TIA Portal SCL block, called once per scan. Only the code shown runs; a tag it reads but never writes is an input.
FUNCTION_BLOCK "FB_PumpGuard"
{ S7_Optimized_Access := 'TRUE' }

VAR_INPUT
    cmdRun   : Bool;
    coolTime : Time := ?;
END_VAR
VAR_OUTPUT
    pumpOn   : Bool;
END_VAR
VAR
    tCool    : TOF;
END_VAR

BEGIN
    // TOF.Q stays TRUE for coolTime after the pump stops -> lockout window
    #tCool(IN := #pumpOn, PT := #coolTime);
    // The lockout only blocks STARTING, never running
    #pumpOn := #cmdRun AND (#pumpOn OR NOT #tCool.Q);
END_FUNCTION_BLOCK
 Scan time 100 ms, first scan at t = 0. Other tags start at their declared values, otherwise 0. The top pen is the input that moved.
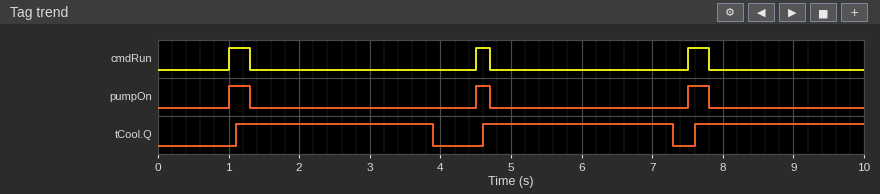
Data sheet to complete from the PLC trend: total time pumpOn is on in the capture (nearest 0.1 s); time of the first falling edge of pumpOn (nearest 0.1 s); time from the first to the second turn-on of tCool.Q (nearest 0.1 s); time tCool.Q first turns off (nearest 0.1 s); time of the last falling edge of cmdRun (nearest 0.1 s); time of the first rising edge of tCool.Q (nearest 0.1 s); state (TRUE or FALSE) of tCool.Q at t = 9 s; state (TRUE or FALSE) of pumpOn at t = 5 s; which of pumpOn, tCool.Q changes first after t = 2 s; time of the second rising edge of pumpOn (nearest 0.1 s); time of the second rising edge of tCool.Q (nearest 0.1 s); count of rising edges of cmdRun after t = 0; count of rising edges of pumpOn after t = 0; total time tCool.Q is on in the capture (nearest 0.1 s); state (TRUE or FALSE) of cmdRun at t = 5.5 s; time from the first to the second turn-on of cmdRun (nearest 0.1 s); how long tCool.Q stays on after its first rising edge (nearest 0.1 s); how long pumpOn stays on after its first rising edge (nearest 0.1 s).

0.8 s
1.3 s
3.5 s
3.9 s
7.8 s
1.1 s
TRUE
FALSE
tCool.Q
4.5 s
4.6 s
3
3
7.9 s
FALSE
3.5 s
2.8 s
0.3 s
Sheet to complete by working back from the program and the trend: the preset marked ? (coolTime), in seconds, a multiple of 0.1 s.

2.5 s
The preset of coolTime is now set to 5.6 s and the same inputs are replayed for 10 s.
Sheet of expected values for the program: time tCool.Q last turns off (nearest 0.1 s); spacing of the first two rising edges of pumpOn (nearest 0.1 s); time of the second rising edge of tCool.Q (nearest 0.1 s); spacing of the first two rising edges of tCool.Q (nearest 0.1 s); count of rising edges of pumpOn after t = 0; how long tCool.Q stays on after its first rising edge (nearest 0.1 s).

7.0 s
6.5 s
7.6 s
6.5 s
2
5.9 s
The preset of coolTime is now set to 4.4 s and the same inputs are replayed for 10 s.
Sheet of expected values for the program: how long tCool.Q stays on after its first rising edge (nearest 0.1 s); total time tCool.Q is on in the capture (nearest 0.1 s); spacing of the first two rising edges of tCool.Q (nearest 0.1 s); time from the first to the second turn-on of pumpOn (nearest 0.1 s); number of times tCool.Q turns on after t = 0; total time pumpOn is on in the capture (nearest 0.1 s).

4.7 s
7.1 s
6.5 s
6.5 s
2
0.6 s
